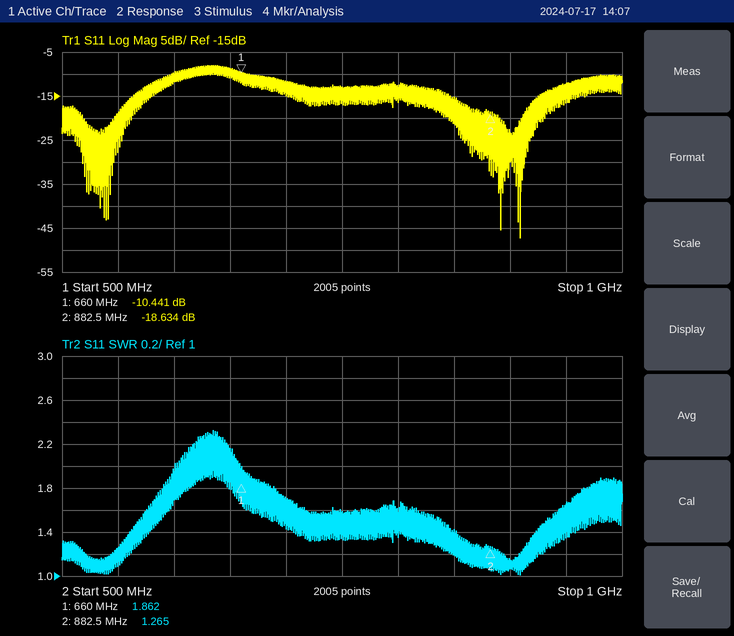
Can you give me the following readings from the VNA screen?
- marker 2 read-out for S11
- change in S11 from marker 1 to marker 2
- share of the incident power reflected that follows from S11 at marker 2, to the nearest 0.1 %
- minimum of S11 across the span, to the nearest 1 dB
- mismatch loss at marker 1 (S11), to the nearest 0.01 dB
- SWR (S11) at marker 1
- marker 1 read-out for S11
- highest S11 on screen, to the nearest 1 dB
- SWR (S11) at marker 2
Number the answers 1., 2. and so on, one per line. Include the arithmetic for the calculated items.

1. -18.634 dB
2. -18.634 − (-10.441) = -8.193 dB
3. 10^(-18.634/10) ≈ 1.4 %
4. -47 dB
5. −10 log10(1 − 10^(-10.441/10)) ≈ 0.41 dB
6. 1.862
7. -10.441 dB
8. -8 dB
9. 1.265
